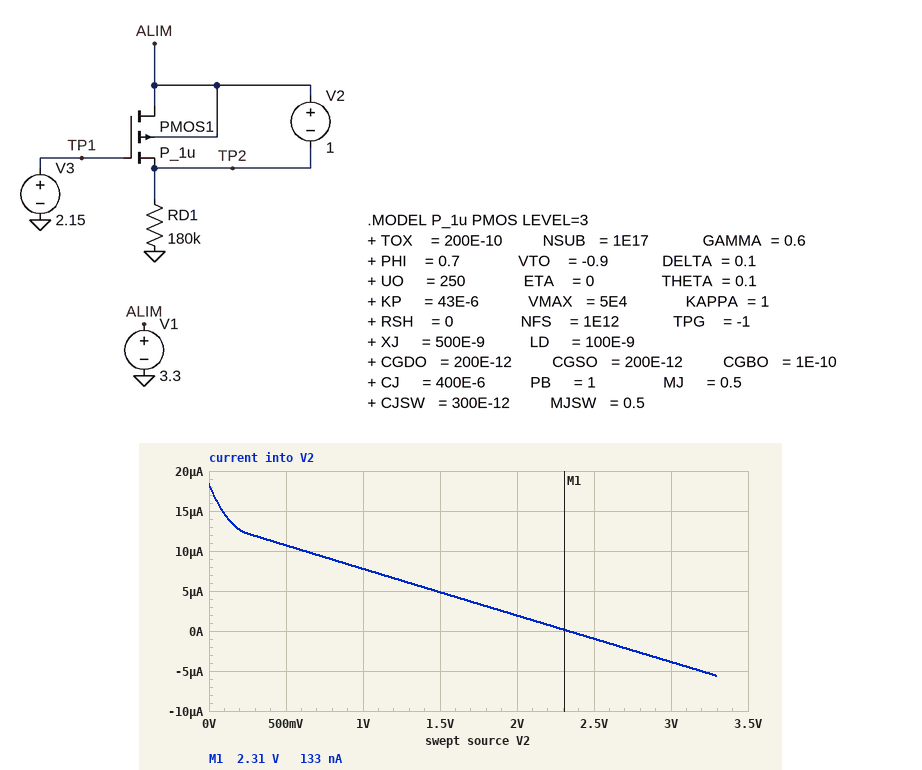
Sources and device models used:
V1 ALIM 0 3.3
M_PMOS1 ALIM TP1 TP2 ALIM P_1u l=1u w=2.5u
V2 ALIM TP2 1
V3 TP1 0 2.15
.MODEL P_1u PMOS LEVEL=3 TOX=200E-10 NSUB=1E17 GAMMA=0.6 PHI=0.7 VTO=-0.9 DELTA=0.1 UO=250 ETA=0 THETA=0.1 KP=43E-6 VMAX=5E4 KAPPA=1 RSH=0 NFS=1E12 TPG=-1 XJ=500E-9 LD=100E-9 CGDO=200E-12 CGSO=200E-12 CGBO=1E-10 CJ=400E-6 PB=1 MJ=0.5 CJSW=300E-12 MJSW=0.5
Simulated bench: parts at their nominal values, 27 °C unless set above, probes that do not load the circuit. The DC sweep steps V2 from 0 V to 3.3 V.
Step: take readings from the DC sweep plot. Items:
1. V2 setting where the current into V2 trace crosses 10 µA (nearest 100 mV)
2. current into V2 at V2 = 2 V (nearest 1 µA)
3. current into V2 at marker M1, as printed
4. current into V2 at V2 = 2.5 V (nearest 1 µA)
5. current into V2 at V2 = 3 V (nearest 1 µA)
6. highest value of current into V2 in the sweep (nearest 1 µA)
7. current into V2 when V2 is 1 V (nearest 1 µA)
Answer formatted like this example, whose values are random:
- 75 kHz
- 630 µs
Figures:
- 600 mV
- 2 µA
- 133 nA
- -1 µA
- -4 µA
- 18 µA
- 8 µA
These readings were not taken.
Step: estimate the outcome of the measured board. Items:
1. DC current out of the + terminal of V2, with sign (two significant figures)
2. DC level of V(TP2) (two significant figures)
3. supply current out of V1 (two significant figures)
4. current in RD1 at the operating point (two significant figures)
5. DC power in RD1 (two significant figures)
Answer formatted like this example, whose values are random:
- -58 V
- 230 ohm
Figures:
- -7.8 µA
- 2.3 V
- 13 µA
- 13 µA
- 29 µW
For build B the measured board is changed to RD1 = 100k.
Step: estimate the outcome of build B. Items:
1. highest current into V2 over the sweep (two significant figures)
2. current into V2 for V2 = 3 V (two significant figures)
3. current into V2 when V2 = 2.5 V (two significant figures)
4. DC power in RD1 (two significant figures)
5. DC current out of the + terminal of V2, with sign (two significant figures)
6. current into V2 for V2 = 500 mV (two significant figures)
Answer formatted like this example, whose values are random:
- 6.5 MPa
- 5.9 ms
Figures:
- 33 µA
- -2.5 µA
- 2.6 µA
- 53 µW
- -18 µA
- 23 µA
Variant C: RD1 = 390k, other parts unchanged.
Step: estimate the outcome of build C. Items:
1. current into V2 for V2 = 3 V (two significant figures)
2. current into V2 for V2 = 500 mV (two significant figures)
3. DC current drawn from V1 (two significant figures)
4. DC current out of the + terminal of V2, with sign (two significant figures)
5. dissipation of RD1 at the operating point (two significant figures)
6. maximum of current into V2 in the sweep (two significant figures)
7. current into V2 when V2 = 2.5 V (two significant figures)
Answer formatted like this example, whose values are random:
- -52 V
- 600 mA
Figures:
- -4.8 µA
- 2.3 µA
- 5.9 µA
- -890 nA
- 14 µW
- 8.5 µA
- -3.4 µA
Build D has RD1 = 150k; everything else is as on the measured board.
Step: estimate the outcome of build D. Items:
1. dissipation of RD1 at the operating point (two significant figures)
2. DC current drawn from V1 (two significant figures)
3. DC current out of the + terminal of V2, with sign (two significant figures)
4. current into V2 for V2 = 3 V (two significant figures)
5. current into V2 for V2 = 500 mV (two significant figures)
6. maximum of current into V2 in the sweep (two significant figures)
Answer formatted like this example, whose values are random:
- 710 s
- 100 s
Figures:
- 35 µW
- 15 µA
- -10 µA
- -3.5 µA
- 14 µA
- 22 µA
